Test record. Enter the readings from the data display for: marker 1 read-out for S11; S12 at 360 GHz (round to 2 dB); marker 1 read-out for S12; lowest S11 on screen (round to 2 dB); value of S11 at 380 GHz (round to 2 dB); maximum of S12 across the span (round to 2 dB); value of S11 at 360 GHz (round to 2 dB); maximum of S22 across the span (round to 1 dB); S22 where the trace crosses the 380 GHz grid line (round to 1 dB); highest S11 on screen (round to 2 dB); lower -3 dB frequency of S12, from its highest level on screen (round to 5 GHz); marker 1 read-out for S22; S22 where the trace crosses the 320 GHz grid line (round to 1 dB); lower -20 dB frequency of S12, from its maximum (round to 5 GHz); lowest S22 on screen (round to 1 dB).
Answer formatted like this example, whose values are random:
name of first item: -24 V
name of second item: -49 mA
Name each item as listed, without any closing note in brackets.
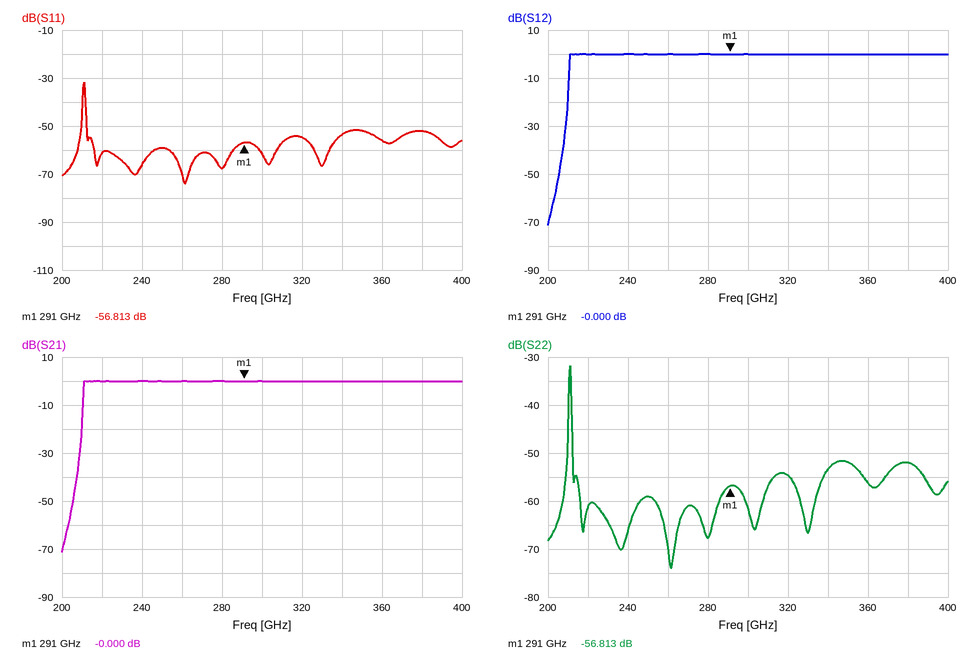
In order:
marker 1 read-out for S11: -56.813 dB
S12 at 360 GHz: 0 dB
marker 1 read-out for S12: -0.000 dB
lowest S11 on screen: -74 dB
value of S11 at 380 GHz: -52 dB
maximum of S12 across the span: 0 dB
value of S11 at 360 GHz: -56 dB
maximum of S22 across the span: -32 dB
S22 where the trace crosses the 380 GHz grid line: -52 dB
highest S11 on screen: -32 dB
lower -3 dB frequency of S12, from its highest level on screen: 210 GHz
marker 1 read-out for S22: -56.813 dB
S22 where the trace crosses the 320 GHz grid line: -55 dB
lower -20 dB frequency of S12, from its maximum: 210 GHz
lowest S22 on screen: -74 dB
